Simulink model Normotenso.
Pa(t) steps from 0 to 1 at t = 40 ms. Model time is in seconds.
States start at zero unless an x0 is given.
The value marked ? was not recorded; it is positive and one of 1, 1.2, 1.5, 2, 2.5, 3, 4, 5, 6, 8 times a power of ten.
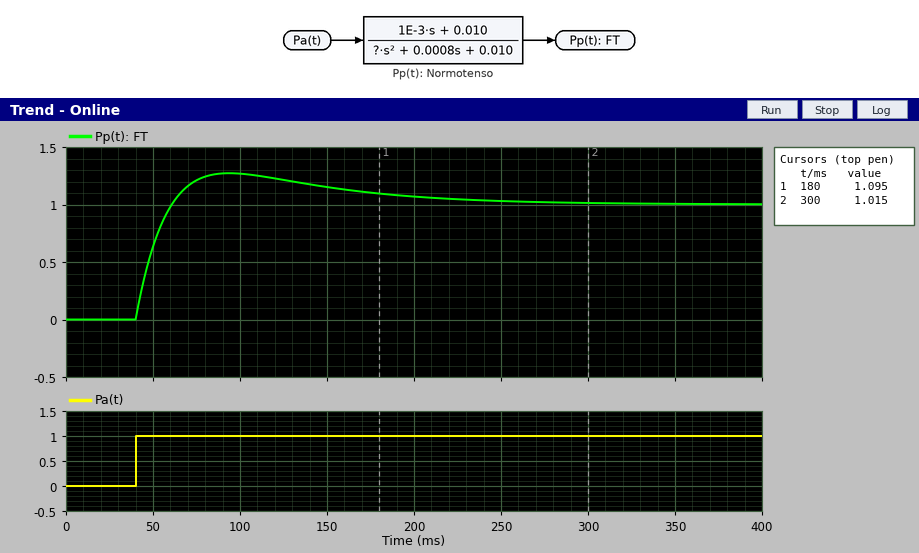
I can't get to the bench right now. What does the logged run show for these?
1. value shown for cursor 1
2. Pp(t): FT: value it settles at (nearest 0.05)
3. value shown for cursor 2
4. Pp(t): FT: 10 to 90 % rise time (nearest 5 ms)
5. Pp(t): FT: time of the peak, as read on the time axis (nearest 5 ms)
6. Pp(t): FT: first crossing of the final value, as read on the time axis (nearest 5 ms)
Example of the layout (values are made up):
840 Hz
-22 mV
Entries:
1.095
1.00
1.015
15 ms
95 ms
60 ms
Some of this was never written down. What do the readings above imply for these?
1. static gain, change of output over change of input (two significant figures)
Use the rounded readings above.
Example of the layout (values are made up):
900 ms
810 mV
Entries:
1.0
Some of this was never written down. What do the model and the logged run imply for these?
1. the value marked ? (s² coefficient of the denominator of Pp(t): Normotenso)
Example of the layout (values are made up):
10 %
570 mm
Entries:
1.2e-05
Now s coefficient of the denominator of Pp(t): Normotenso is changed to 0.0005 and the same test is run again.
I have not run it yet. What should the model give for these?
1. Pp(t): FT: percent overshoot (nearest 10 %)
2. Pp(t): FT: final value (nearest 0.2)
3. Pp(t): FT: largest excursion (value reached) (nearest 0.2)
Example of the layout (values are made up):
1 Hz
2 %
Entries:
70 %
1.0
1.8
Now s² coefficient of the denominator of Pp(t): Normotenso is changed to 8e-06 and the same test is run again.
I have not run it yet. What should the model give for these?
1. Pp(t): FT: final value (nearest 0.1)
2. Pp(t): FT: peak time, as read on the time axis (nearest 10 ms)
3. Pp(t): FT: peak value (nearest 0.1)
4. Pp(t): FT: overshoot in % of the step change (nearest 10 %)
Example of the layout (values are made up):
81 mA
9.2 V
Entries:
1.0
80 ms
1.3
30 %
